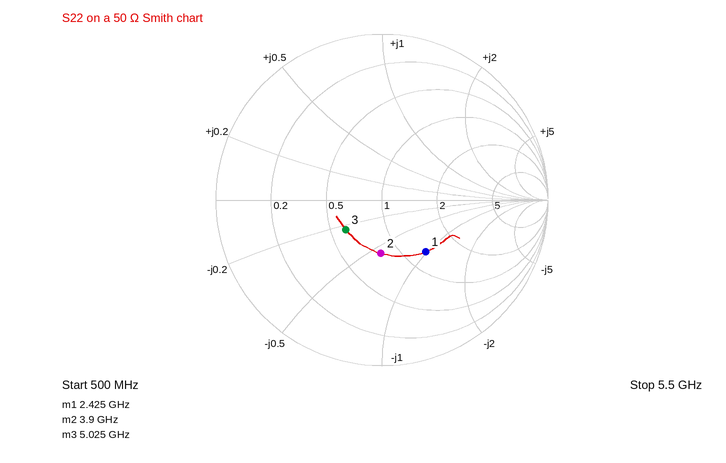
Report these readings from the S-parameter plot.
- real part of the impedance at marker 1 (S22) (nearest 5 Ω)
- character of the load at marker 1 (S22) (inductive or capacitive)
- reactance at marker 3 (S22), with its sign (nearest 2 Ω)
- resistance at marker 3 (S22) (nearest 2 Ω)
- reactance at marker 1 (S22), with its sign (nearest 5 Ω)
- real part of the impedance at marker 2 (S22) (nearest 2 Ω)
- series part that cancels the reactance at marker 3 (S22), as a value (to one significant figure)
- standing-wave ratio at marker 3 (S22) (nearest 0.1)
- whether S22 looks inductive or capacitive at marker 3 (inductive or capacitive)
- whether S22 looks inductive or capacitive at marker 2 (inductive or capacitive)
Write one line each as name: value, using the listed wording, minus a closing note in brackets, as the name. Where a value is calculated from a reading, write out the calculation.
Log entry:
real part of the impedance at marker 1 (S22): 65 Ω
character of the load at marker 1 (S22): capacitive
reactance at marker 3 (S22), with its sign: -12 Ω
resistance at marker 3 (S22): 30 Ω
reactance at marker 1 (S22), with its sign: -50 Ω
real part of the impedance at marker 2 (S22): 40 Ω
series part that cancels the reactance at marker 3 (S22), as a value: L = 12 Ω/(2π × 5.025 GHz) ≈ 380 pH, so 400 pH to one significant figure
standing-wave ratio at marker 3 (S22): 1.8
whether S22 looks inductive or capacitive at marker 3: capacitive
whether S22 looks inductive or capacitive at marker 2: capacitive
